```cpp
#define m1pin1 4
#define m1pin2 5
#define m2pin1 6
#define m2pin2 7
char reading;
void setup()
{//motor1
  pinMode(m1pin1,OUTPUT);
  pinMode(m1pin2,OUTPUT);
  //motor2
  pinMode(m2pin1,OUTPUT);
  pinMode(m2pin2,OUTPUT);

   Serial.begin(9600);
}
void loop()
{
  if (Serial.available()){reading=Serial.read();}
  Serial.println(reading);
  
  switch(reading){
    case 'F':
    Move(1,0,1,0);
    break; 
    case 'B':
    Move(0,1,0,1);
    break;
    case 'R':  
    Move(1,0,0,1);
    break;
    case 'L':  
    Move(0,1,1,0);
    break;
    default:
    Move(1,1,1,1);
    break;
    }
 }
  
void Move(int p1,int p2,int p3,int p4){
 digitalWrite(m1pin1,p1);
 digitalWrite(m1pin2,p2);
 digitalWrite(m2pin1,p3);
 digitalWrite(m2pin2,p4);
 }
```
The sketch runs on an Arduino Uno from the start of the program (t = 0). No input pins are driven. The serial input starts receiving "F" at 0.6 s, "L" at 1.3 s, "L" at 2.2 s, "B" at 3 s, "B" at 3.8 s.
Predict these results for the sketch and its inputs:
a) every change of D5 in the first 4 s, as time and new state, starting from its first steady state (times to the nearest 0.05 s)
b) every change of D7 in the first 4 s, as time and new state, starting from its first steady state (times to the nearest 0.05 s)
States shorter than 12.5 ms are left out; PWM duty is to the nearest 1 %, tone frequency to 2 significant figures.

0 s high; 0.6 s low; 1.3 s high
0 s high; 0.6 s low; 3 s high
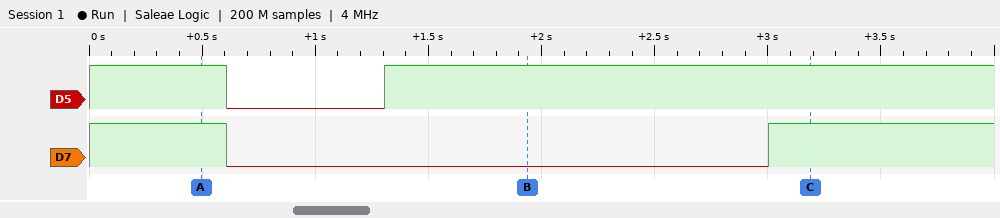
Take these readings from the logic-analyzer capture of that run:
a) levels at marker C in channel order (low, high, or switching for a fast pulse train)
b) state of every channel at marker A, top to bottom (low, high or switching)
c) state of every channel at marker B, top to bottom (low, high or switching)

D5 high, D7 high
D5 high, D7 high
D5 high, D7 low
